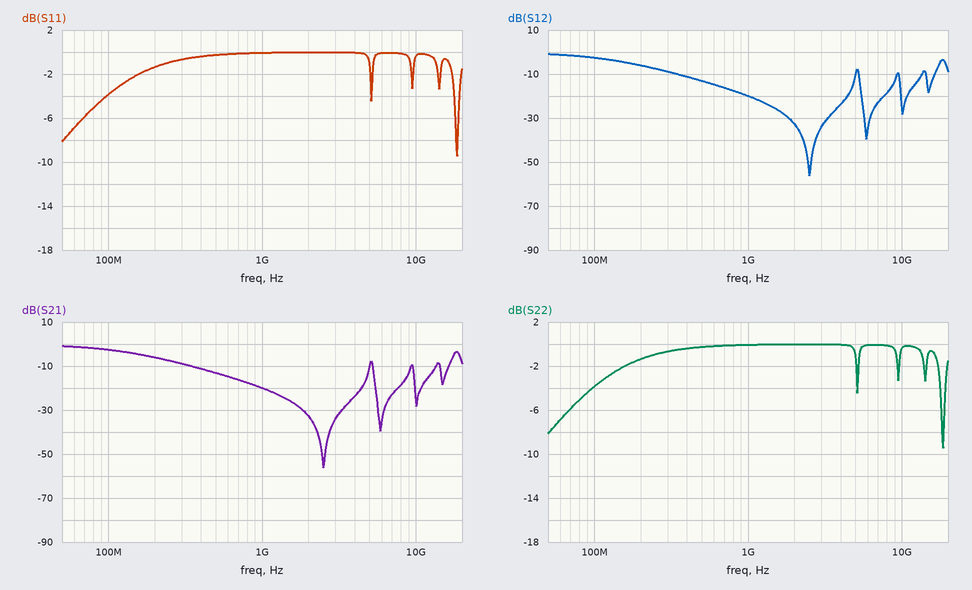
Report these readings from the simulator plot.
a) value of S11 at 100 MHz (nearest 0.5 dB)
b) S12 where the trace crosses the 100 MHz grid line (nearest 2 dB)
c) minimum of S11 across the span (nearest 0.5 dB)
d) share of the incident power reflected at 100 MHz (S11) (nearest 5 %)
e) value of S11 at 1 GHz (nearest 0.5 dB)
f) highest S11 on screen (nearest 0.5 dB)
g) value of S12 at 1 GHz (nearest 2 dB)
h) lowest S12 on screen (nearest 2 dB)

-4.0 dB
-2 dB
-9.5 dB
40 %
0.0 dB
0.0 dB
-20 dB
-56 dB
